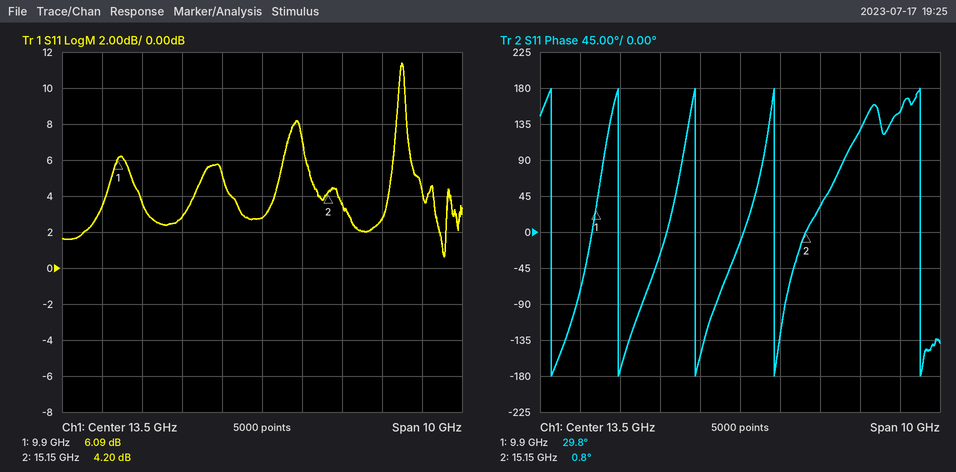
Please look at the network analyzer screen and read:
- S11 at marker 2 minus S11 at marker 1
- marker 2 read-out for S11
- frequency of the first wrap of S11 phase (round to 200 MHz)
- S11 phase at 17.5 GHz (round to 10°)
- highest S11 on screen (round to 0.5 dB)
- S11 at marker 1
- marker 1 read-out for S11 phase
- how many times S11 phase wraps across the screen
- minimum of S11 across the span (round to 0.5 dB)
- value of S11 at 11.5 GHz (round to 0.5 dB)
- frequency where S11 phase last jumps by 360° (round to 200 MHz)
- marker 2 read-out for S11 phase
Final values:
-1.89 dB
4.20 dB
8.8 GHz
150°
11.5 dB
6.09 dB
29.8°
5
0.5 dB
3.0 dB
18.0 GHz
0.8°
